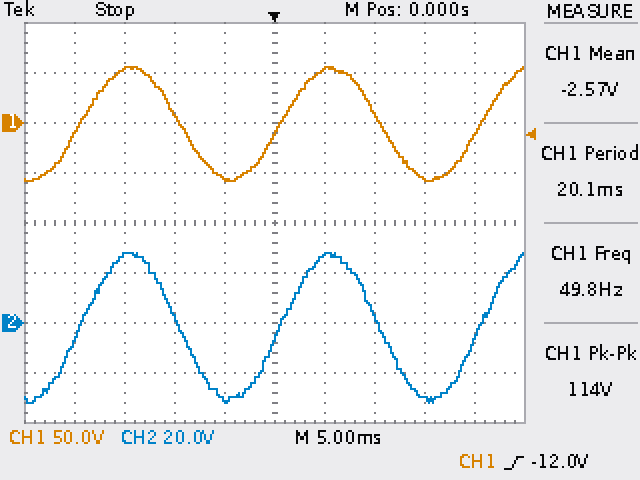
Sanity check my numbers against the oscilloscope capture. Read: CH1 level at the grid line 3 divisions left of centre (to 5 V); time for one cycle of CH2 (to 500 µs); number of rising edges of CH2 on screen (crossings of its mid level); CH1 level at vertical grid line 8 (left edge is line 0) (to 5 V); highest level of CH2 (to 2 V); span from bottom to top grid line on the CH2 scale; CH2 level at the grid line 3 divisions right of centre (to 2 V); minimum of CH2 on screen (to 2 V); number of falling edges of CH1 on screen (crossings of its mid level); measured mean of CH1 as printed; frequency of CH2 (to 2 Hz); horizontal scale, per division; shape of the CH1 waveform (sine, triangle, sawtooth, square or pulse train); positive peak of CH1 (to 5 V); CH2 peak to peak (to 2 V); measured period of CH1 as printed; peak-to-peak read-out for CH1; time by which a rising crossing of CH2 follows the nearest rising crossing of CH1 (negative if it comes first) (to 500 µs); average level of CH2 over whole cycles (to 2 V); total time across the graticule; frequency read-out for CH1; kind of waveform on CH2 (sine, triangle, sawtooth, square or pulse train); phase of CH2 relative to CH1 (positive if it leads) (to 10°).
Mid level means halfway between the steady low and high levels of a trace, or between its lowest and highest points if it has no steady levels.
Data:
55 V
20.0 ms
3
-55 V
28 V
160 V
-30 V
-32 V
2
-2.57 V
50 Hz
5 ms
sine
55 V
60 V
20.1 ms
114 V
0.0 ms
-2 V
50 ms
49.8 Hz
sine
0°
